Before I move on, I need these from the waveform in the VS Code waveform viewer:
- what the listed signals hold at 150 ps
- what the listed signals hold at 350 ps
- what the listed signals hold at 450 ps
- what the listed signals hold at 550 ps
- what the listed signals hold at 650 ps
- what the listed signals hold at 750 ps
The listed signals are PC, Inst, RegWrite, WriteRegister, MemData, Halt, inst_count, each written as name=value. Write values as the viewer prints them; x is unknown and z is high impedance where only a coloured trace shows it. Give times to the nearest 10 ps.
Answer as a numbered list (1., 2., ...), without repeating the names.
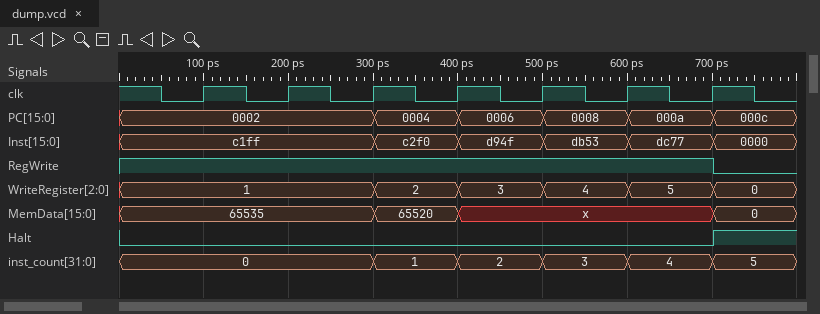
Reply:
1. PC=0002, Inst=c1ff, RegWrite=1, WriteRegister=1, MemData=65535, Halt=0, inst_count=0
2. PC=0004, Inst=c2f0, RegWrite=1, WriteRegister=2, MemData=65520, Halt=0, inst_count=1
3. PC=0006, Inst=d94f, RegWrite=1, WriteRegister=3, MemData=x, Halt=0, inst_count=2
4. PC=0008, Inst=db53, RegWrite=1, WriteRegister=4, MemData=x, Halt=0, inst_count=3
5. PC=000a, Inst=dc77, RegWrite=1, WriteRegister=5, MemData=x, Halt=0, inst_count=4
6. PC=000c, Inst=0000, RegWrite=0, WriteRegister=0, MemData=0, Halt=1, inst_count=5
